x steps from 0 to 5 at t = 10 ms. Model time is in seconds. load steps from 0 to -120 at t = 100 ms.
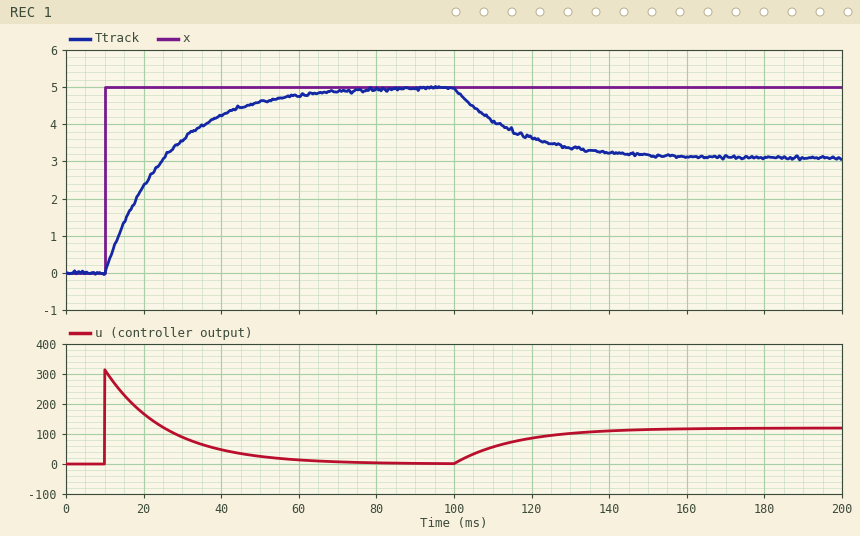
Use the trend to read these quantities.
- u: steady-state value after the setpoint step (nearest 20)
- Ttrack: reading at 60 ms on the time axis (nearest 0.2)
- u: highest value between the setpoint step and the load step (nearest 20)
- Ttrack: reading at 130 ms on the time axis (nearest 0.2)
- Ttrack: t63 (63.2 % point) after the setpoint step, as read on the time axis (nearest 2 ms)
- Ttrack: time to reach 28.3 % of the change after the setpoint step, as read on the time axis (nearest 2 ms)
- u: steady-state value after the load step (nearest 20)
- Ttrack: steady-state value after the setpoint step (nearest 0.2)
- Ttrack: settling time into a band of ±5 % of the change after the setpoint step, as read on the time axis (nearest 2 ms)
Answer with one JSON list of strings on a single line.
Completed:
["0", "4.8", "320", "3.4", "26 ms", "16 ms", "120", "5.0", "58 ms"]
